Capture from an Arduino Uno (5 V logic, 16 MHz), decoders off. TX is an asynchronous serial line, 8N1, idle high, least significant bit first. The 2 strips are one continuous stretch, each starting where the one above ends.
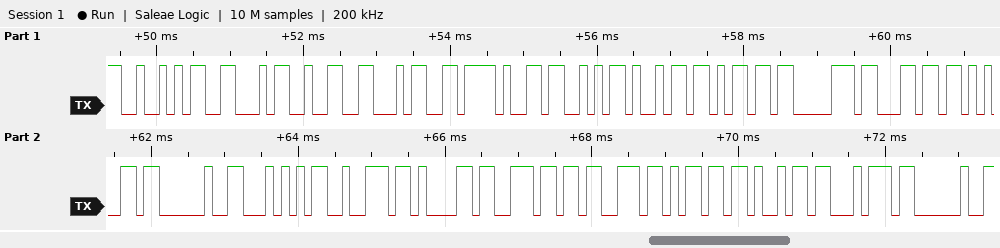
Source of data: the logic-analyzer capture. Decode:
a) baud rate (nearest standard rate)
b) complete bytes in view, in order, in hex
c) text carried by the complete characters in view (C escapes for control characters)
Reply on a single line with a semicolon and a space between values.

9600 baud; 52 46 32 34 2F 53 69 6D 70 6C 65 20 54 72 61 6E 73 6D 69 74 20; "RF24/Simple Transmit "
